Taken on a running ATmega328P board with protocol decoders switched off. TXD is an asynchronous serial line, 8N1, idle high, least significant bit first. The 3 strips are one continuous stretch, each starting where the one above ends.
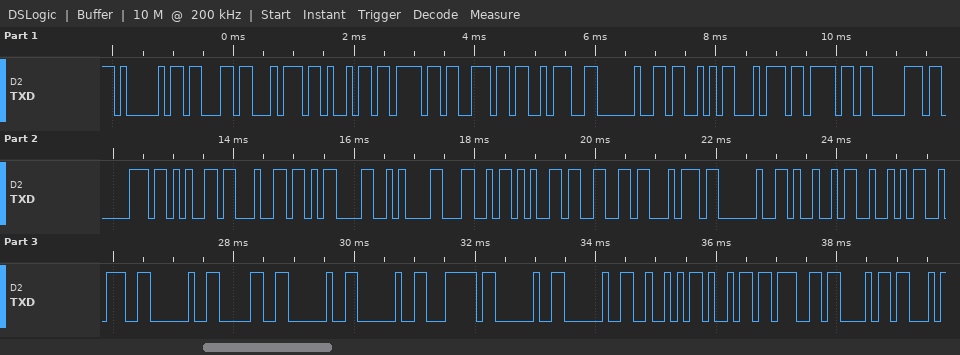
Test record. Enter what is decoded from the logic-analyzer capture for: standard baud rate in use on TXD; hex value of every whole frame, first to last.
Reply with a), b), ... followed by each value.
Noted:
a) 9600 baud
b) 41 63 74 69 6F 6E 3A 20 53 74 6F 70 70 65 64 0D 0A 4C 65 66 74 20 49 52 3A 20 30 20 20 7C 20 20 52 69 67 68
